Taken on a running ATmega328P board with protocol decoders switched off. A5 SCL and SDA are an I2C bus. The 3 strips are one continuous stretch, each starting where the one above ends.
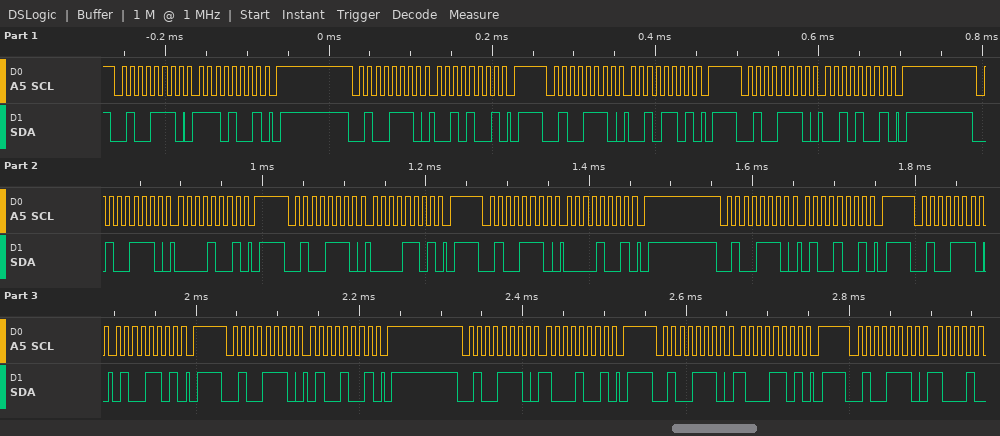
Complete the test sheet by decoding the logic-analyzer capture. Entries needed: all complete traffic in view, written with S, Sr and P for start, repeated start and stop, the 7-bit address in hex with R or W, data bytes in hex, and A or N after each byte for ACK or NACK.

S 27W A E9 A P S 27W A 29 A P S 27W A 2D A P S 27W A 29 A P S 27W A 09 A P S 27W A 0D A P S 27W A 09 A P S 27W A 49 A P S 27W A 4D A P S 27W A 49 A P S 27W A 89 A P S 27W A 8D A P S 27W A
